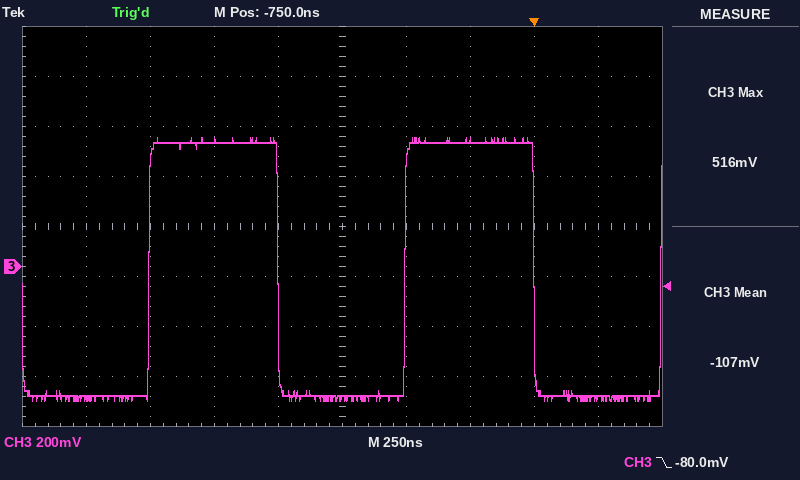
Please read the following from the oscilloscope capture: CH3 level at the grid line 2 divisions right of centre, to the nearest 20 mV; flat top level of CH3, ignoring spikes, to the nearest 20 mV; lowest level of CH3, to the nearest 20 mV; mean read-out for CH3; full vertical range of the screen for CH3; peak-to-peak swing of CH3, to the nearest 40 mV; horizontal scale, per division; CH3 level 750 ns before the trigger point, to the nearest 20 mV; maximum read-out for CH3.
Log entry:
500 mV
500 mV
-540 mV
-107 mV
1.6 V
1.04 V
250 ns
-520 mV
516 mV
